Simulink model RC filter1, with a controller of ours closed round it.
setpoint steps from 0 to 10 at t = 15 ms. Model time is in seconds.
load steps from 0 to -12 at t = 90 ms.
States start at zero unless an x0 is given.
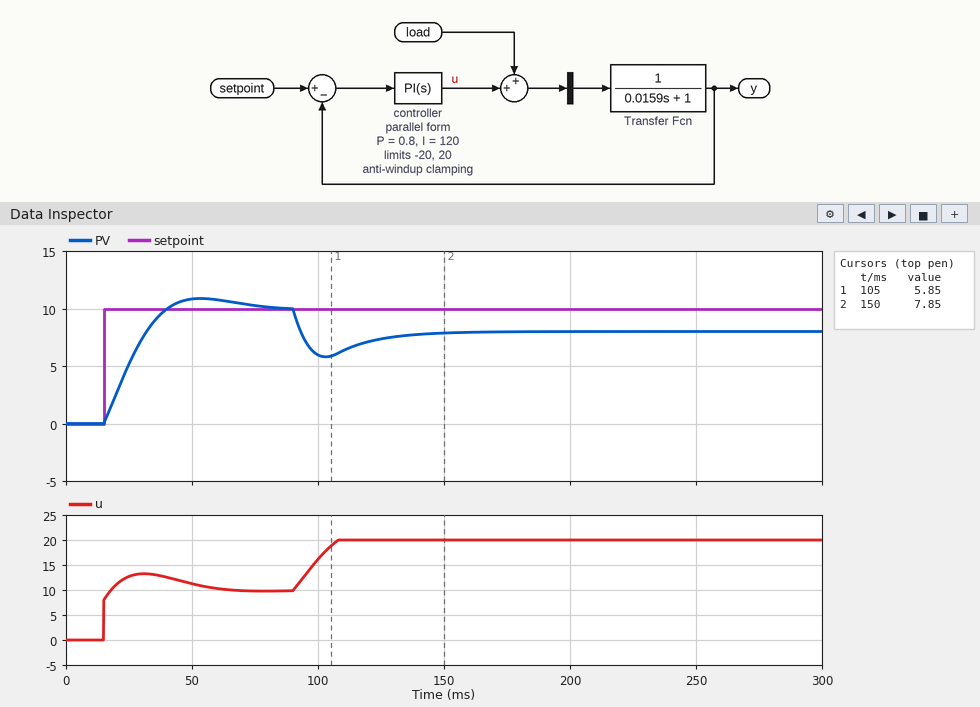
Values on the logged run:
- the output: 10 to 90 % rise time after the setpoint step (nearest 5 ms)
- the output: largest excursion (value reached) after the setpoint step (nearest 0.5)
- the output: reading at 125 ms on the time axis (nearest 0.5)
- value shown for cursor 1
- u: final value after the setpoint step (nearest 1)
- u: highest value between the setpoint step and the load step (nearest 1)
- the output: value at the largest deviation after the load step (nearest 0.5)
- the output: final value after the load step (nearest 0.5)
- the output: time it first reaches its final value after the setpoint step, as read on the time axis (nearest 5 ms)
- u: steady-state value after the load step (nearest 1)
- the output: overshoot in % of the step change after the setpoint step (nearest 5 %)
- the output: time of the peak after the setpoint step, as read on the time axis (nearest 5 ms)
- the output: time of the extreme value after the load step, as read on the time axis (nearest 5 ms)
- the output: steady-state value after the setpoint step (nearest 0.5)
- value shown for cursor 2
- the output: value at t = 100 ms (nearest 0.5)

20 ms
11.0
7.5
5.85
10
13
6.0
8.0
40 ms
20
10 %
55 ms
105 ms
10.0
7.85
6.0
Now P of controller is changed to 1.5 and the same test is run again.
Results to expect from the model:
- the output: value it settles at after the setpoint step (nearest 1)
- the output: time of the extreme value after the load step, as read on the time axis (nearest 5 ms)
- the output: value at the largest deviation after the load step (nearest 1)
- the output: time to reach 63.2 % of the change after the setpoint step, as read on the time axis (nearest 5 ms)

10
100 ms
7
25 ms
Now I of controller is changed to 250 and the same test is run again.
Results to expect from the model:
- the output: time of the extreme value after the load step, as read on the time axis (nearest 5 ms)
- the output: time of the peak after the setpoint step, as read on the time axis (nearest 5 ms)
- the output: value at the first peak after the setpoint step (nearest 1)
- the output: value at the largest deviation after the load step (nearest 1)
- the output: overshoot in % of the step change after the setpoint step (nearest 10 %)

100 ms
40 ms
12
7
20 %
